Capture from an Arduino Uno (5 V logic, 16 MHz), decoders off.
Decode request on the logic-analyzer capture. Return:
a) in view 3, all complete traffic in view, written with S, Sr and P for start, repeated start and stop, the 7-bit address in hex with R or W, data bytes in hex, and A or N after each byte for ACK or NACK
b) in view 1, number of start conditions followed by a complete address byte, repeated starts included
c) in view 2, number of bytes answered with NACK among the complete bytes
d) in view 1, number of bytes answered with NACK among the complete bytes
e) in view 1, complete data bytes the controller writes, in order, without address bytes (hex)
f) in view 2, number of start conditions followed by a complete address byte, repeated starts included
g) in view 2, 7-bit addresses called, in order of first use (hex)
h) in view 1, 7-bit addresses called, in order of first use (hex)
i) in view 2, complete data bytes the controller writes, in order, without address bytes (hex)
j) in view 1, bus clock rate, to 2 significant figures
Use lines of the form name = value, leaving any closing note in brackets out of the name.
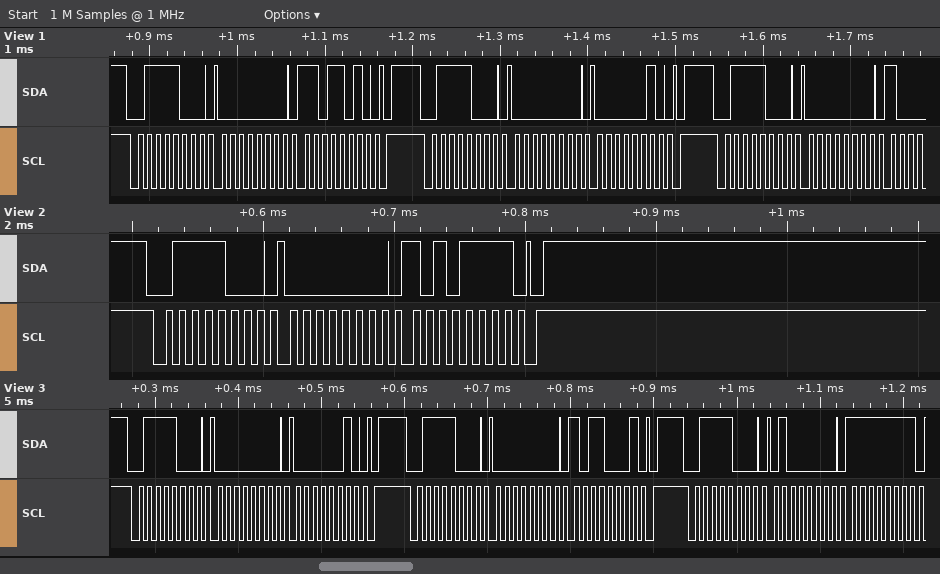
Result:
in view 3, all complete traffic in view, written with S, Sr and P for start, repeated start and stop, the 7-bit address in hex with R or W, data bytes in hex, and A or N after each byte for ACK or NACK = S 3CW A 00 A 02 A P S 3CW A 00 A B1 A P S 3CW A 40 A FF A
in view 1, number of start conditions followed by a complete address byte, repeated starts included = 3
in view 2, number of bytes answered with NACK among the complete bytes = 0
in view 1, number of bytes answered with NACK among the complete bytes = 0
in view 1, complete data bytes the controller writes, in order, without address bytes = 00 DA 00 02 00
in view 2, number of start conditions followed by a complete address byte, repeated starts included = 1
in view 2, 7-bit addresses called, in order of first use = 0x3C
in view 1, 7-bit addresses called, in order of first use = 0x3C
in view 2, complete data bytes the controller writes, in order, without address bytes = 00 AF
in view 1, bus clock rate, to 2 significant figures = 100 kHz
